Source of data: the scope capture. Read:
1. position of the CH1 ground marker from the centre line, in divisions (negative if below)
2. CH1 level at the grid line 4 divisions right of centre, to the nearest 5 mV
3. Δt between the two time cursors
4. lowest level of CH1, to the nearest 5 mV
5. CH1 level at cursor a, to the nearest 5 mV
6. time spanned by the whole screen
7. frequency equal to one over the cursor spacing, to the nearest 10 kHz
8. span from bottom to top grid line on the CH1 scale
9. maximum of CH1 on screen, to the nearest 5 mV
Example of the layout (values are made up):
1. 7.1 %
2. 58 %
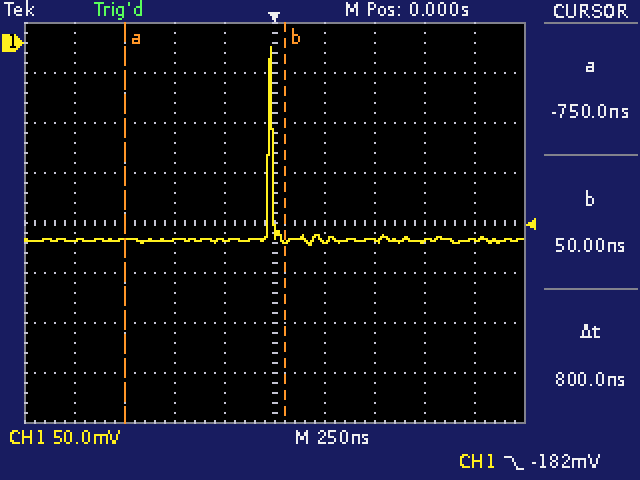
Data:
1. +3.6 div
2. -195 mV
3. 800 ns
4. -200 mV
5. -195 mV
6. 2.5 µs
7. 1.25 MHz
8. 400 mV
9. -5 mV
